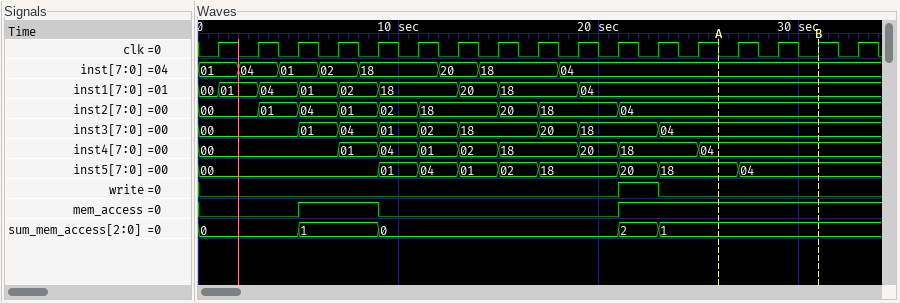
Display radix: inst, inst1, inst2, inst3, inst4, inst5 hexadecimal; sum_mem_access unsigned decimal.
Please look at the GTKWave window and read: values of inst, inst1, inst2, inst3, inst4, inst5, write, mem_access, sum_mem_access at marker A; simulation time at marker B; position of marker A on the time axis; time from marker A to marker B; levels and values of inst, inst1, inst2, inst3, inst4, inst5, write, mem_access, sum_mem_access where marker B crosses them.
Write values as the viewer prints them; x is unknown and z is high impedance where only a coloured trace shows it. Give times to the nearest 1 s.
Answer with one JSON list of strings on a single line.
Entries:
["inst=04, inst1=04, inst2=04, inst3=04, inst4=04, inst5=18, write=0, mem_access=1, sum_mem_access=1", "31 s", "26 s", "5 s", "inst=04, inst1=04, inst2=04, inst3=04, inst4=04, inst5=04, write=0, mem_access=1, sum_mem_access=1"]
